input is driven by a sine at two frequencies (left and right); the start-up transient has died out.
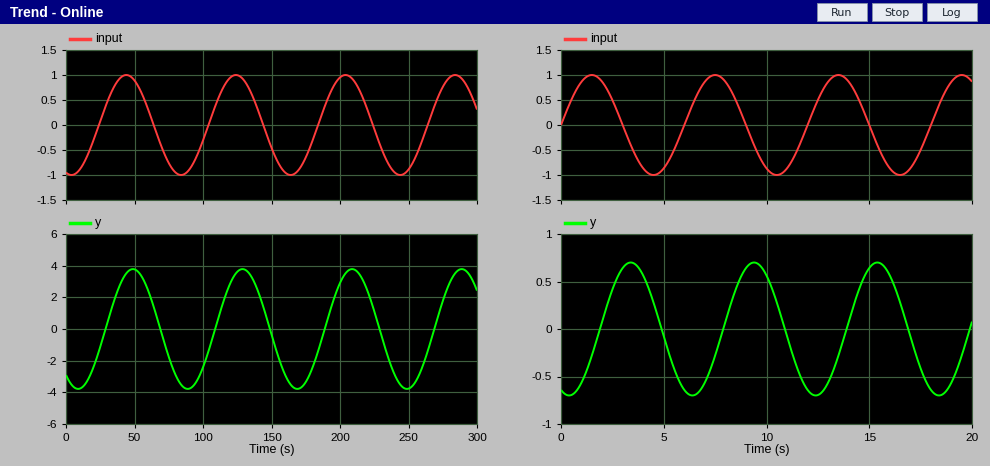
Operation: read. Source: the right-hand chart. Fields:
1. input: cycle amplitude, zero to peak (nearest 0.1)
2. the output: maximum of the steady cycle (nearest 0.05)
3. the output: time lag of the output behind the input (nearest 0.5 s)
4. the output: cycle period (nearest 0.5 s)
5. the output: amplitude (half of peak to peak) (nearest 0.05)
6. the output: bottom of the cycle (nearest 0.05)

1.0
0.70
2.0 s
6.0 s
0.70
-0.70
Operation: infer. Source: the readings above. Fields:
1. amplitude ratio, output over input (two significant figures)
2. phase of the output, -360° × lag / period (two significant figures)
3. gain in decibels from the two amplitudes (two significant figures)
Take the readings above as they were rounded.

0.70
-120°
-3.1 dB
